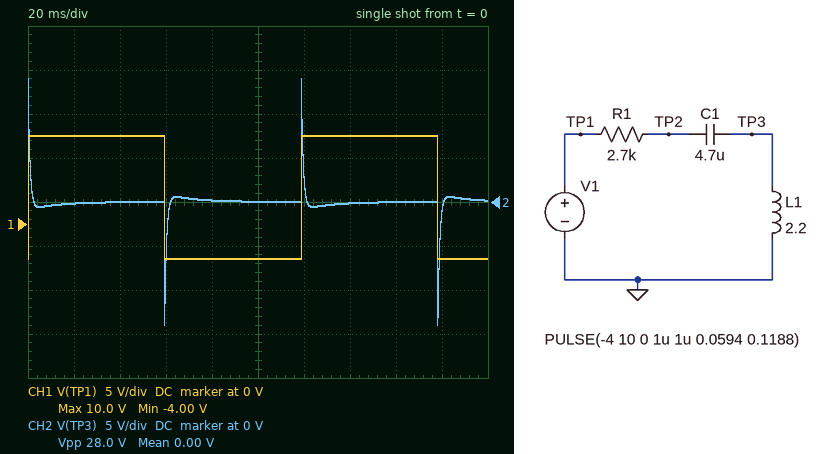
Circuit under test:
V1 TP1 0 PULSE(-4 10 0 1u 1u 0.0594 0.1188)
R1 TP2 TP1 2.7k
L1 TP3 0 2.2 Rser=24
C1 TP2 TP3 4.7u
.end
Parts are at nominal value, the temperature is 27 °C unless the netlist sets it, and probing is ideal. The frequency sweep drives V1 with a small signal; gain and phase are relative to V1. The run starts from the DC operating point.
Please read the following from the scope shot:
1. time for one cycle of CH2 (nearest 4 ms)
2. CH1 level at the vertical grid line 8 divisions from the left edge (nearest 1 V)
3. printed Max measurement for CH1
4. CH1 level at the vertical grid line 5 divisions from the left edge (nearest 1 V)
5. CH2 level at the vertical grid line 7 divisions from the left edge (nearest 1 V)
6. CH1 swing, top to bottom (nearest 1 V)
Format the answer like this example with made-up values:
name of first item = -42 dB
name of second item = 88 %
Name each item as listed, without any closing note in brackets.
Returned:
time for one cycle of CH2 = 120 ms
CH1 level at the vertical grid line 8 divisions from the left edge = 10 V
printed Max measurement for CH1 = 10.0 V
CH1 level at the vertical grid line 5 divisions from the left edge = -4 V
CH2 level at the vertical grid line 7 divisions from the left edge = 0 V
CH1 swing, top to bottom = 14 V
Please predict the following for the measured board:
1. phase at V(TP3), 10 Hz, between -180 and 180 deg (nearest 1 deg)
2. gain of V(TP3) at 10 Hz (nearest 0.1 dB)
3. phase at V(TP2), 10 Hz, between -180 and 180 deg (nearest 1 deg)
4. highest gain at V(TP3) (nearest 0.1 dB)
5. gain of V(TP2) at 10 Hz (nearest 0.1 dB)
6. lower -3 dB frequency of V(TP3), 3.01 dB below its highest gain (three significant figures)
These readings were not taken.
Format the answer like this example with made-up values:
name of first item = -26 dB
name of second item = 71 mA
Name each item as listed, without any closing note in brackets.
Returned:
phase at V(TP3), 10 Hz, between -180 and 180 deg = 130 deg
gain of V(TP3) at 10 Hz = -29.6 dB
phase at V(TP2), 10 Hz, between -180 and 180 deg = -40 deg
highest gain at V(TP3) = 0 dB
gain of V(TP2) at 10 Hz = -2.3 dB
lower -3 dB frequency of V(TP3), 3.01 dB below its highest gain = 185 Hz
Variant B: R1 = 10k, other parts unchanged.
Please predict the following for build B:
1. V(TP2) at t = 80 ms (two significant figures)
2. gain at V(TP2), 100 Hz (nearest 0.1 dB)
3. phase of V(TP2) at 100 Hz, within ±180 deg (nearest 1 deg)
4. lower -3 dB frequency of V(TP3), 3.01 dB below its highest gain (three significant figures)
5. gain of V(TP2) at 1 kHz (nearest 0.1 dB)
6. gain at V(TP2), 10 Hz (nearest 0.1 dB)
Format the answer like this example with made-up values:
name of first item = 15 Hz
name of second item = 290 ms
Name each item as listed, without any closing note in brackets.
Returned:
V(TP2) at t = 80 ms = 2.5 V
gain at V(TP2), 100 Hz = -19.7 dB
phase of V(TP2) at 100 Hz, within ±180 deg = 83 deg
lower -3 dB frequency of V(TP3), 3.01 dB below its highest gain = 722 Hz
gain of V(TP2) at 1 kHz = -1.8 dB
gain at V(TP2), 10 Hz = -10.2 dB
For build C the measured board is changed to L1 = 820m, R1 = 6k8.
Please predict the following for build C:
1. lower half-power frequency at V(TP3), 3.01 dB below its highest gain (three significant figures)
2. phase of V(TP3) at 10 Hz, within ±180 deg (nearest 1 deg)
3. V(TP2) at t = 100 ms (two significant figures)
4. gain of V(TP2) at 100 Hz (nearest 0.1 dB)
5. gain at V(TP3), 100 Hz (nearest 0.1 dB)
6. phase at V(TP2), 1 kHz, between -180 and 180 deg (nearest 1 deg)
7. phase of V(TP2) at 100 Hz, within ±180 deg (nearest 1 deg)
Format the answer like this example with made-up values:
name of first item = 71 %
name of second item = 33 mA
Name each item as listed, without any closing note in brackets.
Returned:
lower half-power frequency at V(TP3), 3.01 dB below its highest gain = 1.32 kHz
phase of V(TP3) at 10 Hz, within ±180 deg = 91 deg
V(TP2) at t = 100 ms = -670 mV
gain of V(TP2) at 100 Hz = -31.7 dB
gain at V(TP3), 100 Hz = -22.4 dB
phase at V(TP2), 1 kHz, between -180 and 180 deg = 53 deg
phase of V(TP2) at 100 Hz, within ±180 deg = 81 deg
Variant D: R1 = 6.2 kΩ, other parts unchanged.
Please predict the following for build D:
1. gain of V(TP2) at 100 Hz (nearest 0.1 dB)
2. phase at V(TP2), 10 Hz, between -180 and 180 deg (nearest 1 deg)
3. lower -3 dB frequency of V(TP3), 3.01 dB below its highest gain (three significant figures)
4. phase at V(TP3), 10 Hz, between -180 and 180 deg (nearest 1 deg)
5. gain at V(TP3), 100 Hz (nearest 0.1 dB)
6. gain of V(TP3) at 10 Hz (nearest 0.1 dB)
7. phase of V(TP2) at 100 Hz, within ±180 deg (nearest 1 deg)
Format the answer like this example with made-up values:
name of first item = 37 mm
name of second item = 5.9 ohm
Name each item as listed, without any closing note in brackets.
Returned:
gain of V(TP2) at 100 Hz = -15.6 dB
phase at V(TP2), 10 Hz, between -180 and 180 deg = -62 deg
lower -3 dB frequency of V(TP3), 3.01 dB below its highest gain = 445 Hz
phase at V(TP3), 10 Hz, between -180 and 180 deg = 108 deg
gain at V(TP3), 100 Hz = -13.2 dB
gain of V(TP3) at 10 Hz = -34.0 dB
phase of V(TP2) at 100 Hz, within ±180 deg = 79 deg
